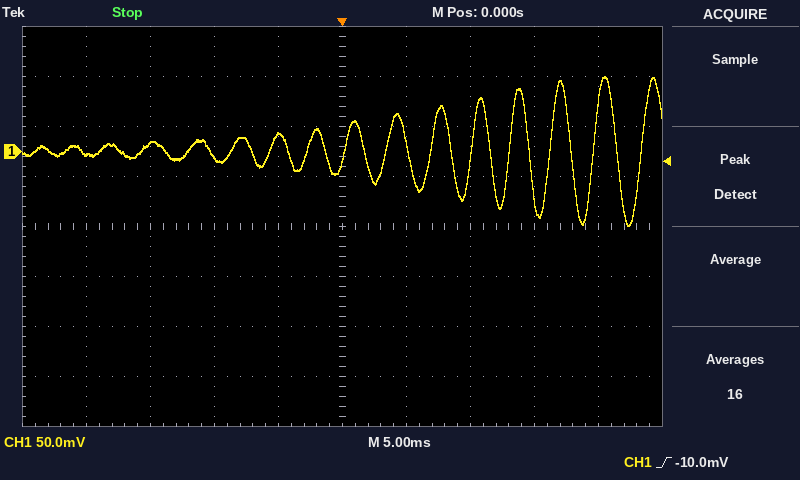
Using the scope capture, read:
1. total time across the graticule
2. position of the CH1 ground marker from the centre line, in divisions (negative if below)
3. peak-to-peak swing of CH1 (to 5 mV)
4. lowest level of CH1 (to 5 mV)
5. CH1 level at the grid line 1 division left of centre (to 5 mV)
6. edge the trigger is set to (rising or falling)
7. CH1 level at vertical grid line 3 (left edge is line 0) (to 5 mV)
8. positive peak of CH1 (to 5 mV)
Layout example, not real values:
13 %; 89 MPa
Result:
50 ms; +1.5 div; 150 mV; -75 mV; 15 mV; rising; -5 mV; 75 mV
